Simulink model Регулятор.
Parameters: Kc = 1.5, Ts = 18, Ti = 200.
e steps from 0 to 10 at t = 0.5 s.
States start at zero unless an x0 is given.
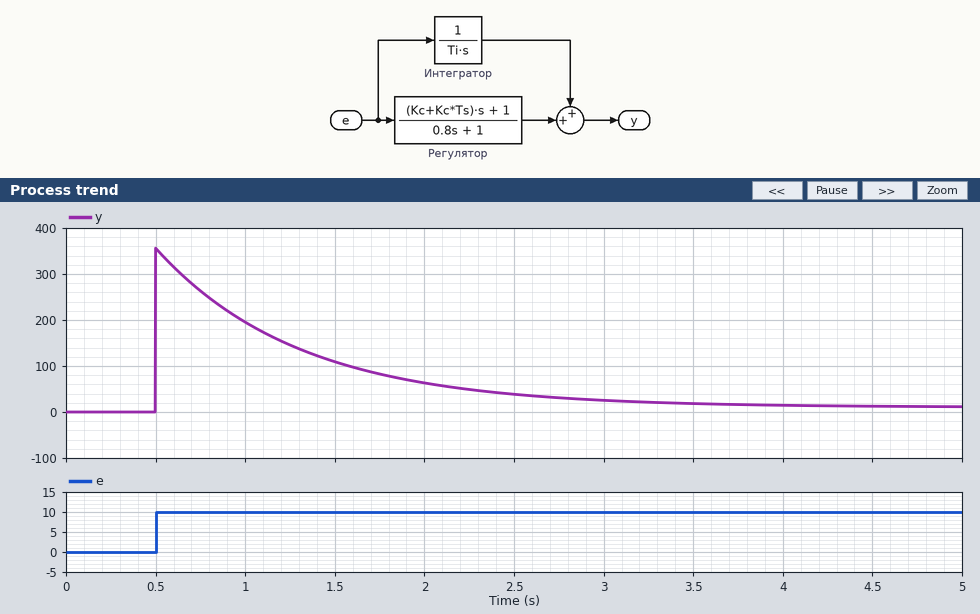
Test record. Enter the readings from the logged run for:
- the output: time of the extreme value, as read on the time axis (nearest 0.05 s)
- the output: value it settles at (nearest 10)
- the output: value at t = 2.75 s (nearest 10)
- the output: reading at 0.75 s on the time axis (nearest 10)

0.50 s
10
30
260
